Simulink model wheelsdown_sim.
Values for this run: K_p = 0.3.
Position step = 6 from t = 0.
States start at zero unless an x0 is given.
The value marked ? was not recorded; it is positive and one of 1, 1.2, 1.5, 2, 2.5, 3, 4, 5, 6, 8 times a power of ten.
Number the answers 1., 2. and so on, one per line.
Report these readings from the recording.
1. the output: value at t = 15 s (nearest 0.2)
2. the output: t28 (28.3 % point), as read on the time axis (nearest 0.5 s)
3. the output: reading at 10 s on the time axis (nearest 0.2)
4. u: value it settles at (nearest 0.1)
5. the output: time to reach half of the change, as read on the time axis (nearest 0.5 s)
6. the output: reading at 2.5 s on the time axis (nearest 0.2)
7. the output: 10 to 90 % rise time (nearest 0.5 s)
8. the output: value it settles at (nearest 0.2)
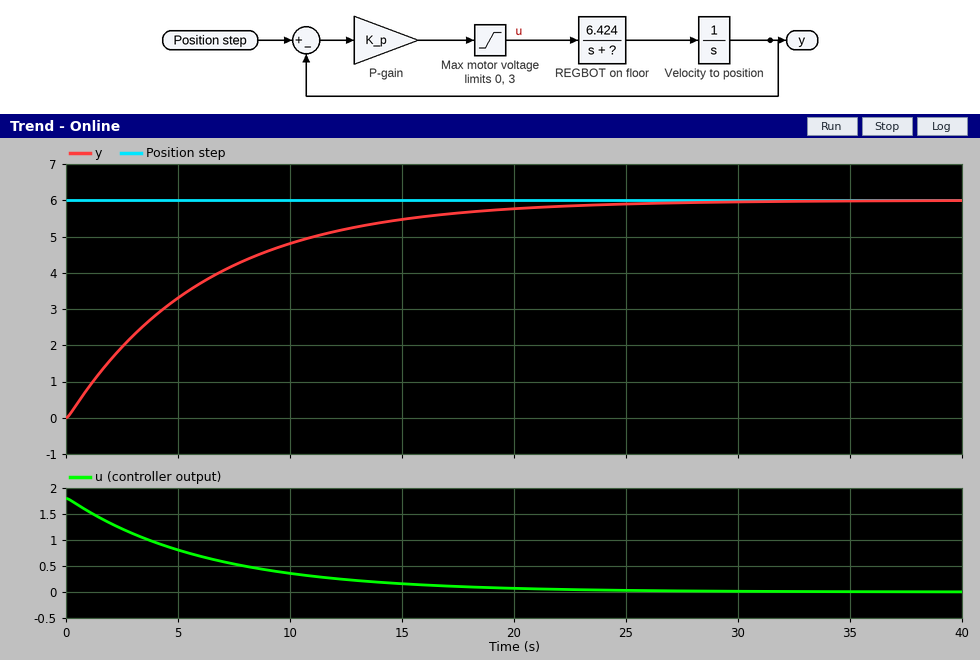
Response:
1. 5.4
2. 2.0 s
3. 4.8
4. 0.0
5. 4.5 s
6. 2.0
7. 13.5 s
8. 6.0
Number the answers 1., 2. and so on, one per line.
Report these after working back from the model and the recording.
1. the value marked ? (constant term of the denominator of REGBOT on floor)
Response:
1. 12
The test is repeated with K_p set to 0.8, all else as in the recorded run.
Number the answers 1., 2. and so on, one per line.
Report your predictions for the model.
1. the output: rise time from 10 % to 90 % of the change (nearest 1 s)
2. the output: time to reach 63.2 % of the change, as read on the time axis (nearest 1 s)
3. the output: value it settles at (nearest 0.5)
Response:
1. 5 s
2. 3 s
3. 6.0
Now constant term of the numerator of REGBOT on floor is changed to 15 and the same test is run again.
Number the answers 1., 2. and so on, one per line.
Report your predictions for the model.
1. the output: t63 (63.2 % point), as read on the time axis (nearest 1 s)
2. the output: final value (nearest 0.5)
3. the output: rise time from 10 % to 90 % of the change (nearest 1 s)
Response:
1. 3 s
2. 6.0
3. 6 s
